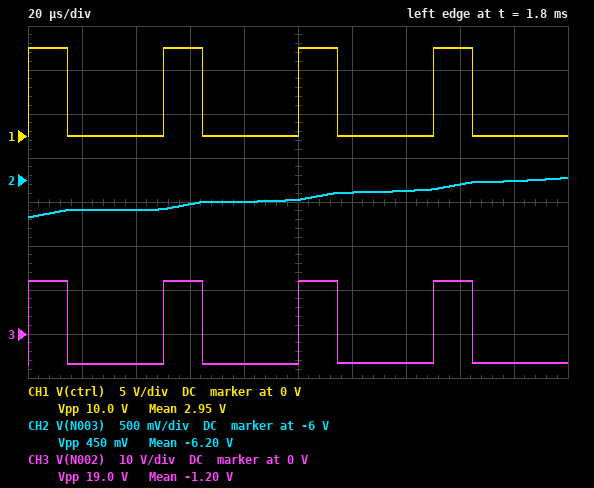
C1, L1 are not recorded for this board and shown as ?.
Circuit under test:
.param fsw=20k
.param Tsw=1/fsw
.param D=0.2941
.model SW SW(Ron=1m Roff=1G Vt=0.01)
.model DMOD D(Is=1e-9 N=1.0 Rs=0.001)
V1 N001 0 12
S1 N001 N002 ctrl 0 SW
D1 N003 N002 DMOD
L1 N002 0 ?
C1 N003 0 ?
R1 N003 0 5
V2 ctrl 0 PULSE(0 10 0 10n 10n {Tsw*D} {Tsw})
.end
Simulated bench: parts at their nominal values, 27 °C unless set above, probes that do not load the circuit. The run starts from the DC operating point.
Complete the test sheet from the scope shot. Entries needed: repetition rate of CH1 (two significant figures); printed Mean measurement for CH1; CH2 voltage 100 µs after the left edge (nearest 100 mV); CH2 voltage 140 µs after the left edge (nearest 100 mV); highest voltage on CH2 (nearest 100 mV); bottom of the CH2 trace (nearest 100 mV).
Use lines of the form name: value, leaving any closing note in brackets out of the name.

repetition rate of CH1: 20 kHz
printed Mean measurement for CH1: 2.95 V
CH2 voltage 100 µs after the left edge: -6.2 V
CH2 voltage 140 µs after the left edge: -6.1 V
highest voltage on CH2: -6.0 V
bottom of the CH2 trace: -6.4 V
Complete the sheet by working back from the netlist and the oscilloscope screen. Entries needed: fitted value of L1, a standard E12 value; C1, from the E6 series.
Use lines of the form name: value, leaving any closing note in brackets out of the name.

fitted value of L1, a standard E12 value: 560 µH
C1, from the E6 series: 220 µF
